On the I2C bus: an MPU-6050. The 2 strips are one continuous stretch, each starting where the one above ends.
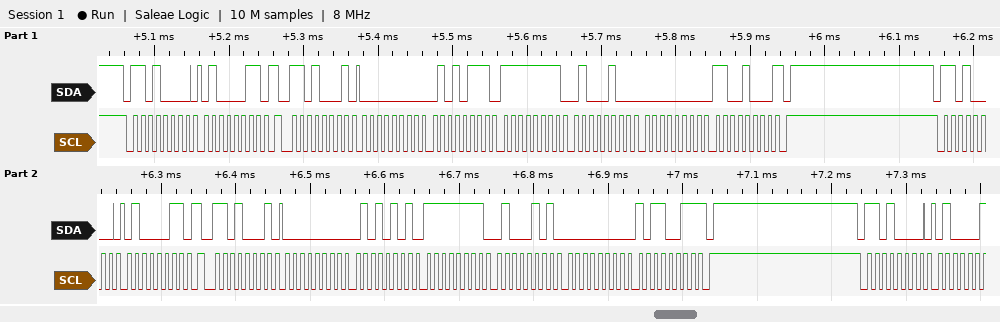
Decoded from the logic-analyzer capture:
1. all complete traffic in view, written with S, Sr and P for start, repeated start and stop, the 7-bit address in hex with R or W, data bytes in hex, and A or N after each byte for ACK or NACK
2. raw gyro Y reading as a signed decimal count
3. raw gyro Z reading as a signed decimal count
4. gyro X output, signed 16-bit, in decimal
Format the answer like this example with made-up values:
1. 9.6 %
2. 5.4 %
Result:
1. S 68W A 43 A Sr 68R A 00 A 57 A FF A 44 A 00 A C8 N P S 68W A 43 A Sr 68R A 00 A 55 A FF A 45 A 00 A B3 N P S 68W A
2. -188
3. 200
4. 87
